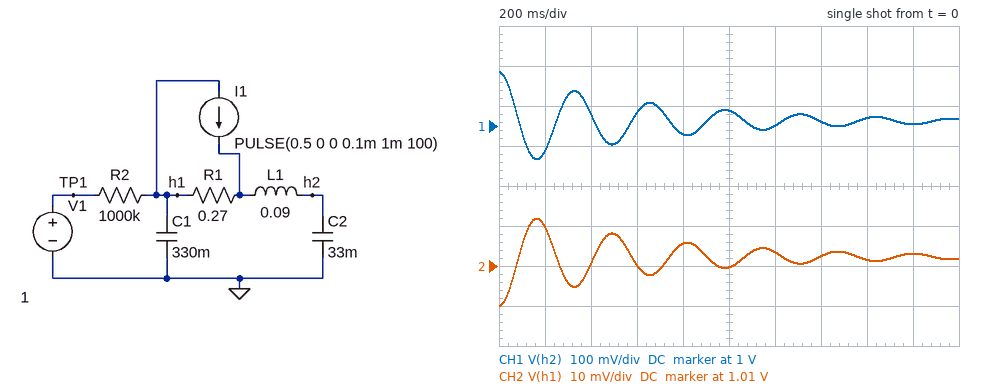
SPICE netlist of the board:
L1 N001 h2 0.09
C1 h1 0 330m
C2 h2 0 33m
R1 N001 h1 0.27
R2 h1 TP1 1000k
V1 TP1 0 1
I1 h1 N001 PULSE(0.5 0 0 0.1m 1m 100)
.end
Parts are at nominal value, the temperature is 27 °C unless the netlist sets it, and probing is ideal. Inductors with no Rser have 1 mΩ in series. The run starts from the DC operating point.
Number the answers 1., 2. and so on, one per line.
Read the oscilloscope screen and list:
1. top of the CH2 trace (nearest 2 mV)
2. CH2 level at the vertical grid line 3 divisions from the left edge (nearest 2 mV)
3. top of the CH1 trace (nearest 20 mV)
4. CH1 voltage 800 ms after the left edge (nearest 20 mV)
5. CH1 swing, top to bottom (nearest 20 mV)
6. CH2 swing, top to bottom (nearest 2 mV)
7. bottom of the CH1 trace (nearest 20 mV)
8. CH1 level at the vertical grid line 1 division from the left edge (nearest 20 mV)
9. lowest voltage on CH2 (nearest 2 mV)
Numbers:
1. 1.022 V
2. 1.010 V
3. 1.14 V
4. 980 mV
5. 220 mV
6. 22 mV
7. 920 mV
8. 940 mV
9. 1.000 V
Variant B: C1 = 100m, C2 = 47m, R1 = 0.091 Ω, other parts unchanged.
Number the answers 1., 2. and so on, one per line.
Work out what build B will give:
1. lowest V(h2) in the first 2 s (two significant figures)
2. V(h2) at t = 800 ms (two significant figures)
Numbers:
1. 990 mV
2. 1.0 V
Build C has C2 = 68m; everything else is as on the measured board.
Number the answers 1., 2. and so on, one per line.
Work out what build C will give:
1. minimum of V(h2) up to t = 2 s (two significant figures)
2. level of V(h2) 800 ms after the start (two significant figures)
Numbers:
1. 940 mV
2. 1.0 V
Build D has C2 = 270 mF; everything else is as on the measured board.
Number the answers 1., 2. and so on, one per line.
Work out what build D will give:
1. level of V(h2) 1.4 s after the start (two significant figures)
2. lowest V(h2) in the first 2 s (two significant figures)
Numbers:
1. 1.1 V
2. 1.0 V
